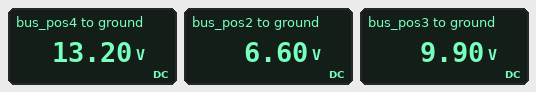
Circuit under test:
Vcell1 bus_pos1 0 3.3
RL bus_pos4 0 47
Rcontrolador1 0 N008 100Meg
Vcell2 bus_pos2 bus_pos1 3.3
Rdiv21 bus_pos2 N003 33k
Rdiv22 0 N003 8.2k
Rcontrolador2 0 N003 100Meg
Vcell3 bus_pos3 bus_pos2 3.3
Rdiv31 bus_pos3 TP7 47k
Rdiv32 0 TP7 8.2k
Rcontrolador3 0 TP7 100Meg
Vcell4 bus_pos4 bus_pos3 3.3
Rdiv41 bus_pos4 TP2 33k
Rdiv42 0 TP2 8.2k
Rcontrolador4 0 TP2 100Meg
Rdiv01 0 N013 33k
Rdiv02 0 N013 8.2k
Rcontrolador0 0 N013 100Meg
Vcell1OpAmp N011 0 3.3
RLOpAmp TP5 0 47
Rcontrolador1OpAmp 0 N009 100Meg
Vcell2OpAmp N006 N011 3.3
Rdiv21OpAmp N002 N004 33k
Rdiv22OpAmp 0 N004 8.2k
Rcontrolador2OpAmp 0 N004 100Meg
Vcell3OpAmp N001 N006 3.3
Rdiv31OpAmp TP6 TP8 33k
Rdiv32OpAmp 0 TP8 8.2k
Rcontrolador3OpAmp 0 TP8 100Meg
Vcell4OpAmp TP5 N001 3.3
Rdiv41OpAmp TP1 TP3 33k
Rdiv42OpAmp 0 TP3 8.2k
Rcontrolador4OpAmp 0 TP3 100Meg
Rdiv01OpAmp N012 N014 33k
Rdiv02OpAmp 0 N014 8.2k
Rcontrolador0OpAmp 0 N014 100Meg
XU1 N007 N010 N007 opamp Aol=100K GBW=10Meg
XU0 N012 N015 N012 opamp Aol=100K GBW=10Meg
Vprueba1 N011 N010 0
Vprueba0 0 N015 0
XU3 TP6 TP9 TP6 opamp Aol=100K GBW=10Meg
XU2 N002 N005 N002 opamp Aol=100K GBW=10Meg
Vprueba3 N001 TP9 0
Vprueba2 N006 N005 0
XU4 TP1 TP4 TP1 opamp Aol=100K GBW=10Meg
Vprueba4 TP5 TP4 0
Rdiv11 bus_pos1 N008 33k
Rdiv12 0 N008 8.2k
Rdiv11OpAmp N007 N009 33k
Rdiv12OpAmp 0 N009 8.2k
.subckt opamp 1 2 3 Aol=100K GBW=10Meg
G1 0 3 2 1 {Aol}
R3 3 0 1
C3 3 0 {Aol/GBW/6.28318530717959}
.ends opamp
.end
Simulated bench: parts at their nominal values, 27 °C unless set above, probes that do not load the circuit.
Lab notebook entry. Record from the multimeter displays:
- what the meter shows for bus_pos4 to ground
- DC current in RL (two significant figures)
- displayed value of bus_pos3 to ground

13.20 V
280 mA
9.90 V
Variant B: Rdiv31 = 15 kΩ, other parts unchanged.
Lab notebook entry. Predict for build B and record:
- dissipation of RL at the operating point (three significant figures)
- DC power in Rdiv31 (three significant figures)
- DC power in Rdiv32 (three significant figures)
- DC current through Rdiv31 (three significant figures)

3.71 W
2.73 mW
1.49 mW
427 µA
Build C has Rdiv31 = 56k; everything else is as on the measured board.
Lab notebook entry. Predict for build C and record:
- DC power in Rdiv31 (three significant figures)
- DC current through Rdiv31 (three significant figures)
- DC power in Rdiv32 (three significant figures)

1.33 mW
154 µA
195 µW
